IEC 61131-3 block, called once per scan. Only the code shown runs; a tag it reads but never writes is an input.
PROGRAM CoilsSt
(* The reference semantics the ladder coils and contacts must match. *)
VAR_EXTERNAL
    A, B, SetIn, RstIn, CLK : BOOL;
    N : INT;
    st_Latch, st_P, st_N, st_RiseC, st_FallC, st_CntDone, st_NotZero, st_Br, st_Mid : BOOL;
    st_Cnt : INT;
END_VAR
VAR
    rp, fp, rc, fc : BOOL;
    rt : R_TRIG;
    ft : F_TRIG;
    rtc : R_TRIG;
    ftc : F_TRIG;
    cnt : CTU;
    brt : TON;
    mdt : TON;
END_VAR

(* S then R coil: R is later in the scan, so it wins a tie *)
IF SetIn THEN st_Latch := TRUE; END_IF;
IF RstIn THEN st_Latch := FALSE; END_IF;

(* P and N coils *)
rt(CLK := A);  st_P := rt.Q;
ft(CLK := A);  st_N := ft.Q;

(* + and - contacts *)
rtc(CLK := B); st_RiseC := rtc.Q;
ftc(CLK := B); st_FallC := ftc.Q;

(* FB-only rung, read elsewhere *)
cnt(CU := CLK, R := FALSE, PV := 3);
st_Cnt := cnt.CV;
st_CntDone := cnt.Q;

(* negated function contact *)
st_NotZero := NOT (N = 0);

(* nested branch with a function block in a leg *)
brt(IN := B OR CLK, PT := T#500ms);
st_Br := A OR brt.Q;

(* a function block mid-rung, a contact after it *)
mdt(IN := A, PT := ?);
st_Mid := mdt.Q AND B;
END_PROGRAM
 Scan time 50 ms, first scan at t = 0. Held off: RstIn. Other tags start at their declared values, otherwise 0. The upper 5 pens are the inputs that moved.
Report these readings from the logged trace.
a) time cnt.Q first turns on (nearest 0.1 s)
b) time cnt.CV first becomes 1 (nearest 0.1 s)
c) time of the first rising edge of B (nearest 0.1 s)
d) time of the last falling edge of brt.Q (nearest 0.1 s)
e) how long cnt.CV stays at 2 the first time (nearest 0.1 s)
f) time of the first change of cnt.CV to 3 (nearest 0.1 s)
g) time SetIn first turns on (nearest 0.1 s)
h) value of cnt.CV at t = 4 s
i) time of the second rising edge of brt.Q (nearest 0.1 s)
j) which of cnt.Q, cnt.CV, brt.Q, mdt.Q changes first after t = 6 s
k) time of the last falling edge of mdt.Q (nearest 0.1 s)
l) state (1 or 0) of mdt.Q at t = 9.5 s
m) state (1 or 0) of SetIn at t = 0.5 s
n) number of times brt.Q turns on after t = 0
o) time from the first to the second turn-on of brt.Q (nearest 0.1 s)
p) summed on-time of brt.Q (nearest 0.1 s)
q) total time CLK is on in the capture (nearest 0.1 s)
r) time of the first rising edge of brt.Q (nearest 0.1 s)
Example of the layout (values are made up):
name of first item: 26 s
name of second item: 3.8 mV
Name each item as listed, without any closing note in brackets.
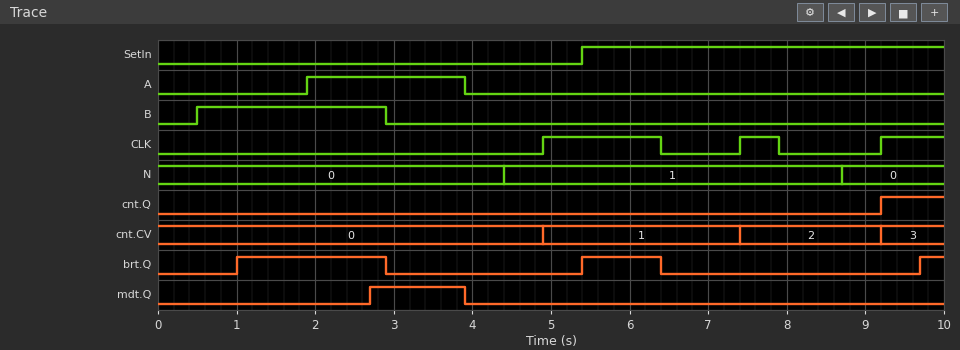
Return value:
time cnt.Q first turns on: 9.2 s
time cnt.CV first becomes 1: 4.9 s
time of the first rising edge of B: 0.5 s
time of the last falling edge of brt.Q: 6.4 s
how long cnt.CV stays at 2 the first time: 1.8 s
time of the first change of cnt.CV to 3: 9.2 s
time SetIn first turns on: 5.4 s
value of cnt.CV at t = 4 s: 0
time of the second rising edge of brt.Q: 5.4 s
which of cnt.Q, cnt.CV, brt.Q, mdt.Q changes first after t = 6 s: brt.Q
time of the last falling edge of mdt.Q: 3.9 s
state (1 or 0) of mdt.Q at t = 9.5 s: 0
state (1 or 0) of SetIn at t = 0.5 s: 0
number of times brt.Q turns on after t = 0: 3
time from the first to the second turn-on of brt.Q: 4.4 s
summed on-time of brt.Q: 3.2 s
total time CLK is on in the capture: 2.8 s
time of the first rising edge of brt.Q: 1.0 s
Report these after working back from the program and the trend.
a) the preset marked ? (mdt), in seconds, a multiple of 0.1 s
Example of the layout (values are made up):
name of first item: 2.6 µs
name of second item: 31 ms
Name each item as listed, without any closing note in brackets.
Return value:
the preset marked ? (mdt), in seconds, a multiple of 0.1 s: 0.8 s
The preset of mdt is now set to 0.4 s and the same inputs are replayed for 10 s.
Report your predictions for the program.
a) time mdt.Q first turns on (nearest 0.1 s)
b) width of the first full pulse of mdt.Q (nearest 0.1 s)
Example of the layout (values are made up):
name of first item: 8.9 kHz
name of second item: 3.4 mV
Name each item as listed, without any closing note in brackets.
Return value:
time mdt.Q first turns on: 2.3 s
width of the first full pulse of mdt.Q: 1.6 s
